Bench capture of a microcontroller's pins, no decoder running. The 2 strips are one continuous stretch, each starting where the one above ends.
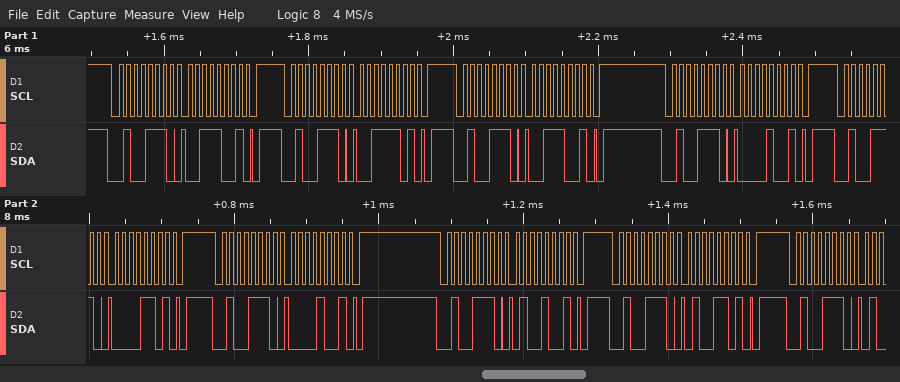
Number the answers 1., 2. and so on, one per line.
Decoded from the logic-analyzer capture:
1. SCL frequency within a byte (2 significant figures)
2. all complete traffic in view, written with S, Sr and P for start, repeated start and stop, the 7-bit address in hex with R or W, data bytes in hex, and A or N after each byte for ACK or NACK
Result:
1. 100 kHz
2. S 27W A 39 A P S 27W A 3D A P S 27W A 39 A P S 27W A 09 A P S 27W A 0D A P S 27W A 09 A P S 27W A 49 A P S 27W A 4D A P S 27W A
